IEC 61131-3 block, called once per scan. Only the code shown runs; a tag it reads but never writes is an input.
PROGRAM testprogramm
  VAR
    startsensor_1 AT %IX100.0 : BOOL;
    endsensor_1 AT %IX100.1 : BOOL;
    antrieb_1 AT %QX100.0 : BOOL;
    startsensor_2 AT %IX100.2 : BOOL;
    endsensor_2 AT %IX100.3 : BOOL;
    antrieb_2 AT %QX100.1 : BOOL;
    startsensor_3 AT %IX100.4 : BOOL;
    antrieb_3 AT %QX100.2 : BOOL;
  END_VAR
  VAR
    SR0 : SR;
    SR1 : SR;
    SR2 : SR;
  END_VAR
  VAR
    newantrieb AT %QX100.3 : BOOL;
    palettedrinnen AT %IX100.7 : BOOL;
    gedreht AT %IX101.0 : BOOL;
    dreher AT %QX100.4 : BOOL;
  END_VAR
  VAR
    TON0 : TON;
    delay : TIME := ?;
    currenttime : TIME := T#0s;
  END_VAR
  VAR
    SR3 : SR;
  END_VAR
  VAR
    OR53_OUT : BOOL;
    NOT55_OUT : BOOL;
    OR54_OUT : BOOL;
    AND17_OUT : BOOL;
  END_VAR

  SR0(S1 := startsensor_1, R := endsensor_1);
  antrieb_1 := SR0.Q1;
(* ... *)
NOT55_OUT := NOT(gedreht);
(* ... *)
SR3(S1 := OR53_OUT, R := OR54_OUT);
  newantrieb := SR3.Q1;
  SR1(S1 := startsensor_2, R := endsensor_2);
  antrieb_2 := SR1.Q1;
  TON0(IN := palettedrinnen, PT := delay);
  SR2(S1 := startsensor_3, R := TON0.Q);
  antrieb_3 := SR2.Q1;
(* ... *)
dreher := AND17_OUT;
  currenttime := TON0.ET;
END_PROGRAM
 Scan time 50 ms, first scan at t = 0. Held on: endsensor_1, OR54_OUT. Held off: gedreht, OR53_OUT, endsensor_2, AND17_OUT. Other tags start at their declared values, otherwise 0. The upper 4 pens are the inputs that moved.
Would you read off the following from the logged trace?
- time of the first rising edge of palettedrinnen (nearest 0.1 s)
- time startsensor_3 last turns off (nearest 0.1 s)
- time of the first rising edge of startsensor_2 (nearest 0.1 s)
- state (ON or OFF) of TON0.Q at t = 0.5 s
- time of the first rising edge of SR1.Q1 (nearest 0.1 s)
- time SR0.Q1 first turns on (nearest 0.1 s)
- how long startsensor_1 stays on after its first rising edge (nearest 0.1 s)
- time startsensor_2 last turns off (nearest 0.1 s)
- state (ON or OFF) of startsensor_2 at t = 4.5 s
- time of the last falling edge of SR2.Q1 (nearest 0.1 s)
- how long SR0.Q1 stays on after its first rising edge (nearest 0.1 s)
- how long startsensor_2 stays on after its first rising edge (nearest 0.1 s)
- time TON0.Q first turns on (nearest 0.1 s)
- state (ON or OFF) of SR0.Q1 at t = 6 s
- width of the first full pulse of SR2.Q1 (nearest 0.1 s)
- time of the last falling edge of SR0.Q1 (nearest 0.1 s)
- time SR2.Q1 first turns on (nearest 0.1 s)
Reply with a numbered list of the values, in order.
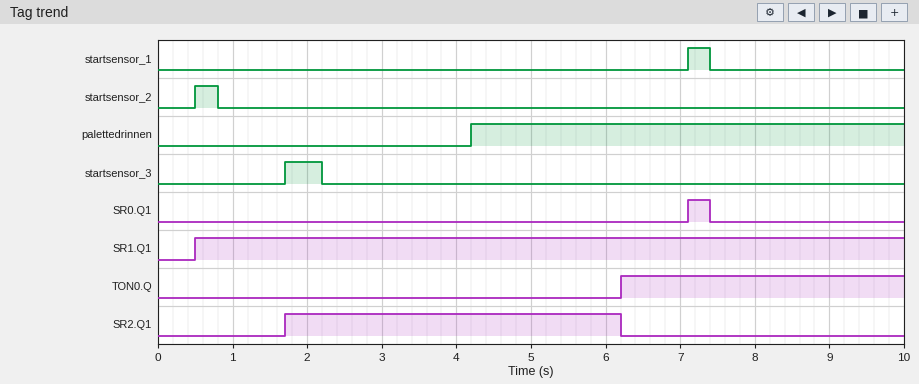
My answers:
1. 4.2 s
2. 2.2 s
3. 0.5 s
4. OFF
5. 0.5 s
6. 7.1 s
7. 0.3 s
8. 0.8 s
9. OFF
10. 6.2 s
11. 0.3 s
12. 0.3 s
13. 6.2 s
14. OFF
15. 4.5 s
16. 7.4 s
17. 1.7 s
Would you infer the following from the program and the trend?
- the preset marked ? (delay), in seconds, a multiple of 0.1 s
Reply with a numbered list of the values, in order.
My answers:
1. 2.0 s
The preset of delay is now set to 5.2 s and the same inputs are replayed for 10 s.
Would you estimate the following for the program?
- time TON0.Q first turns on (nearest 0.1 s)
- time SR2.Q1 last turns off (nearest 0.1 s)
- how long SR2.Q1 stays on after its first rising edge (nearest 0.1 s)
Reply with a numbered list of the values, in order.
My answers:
1. 9.4 s
2. 9.4 s
3. 7.7 s
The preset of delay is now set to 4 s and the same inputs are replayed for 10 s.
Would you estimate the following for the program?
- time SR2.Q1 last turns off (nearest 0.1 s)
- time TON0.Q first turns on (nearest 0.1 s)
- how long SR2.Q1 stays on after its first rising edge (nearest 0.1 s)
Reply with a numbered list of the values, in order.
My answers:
1. 8.2 s
2. 8.2 s
3. 6.5 s
